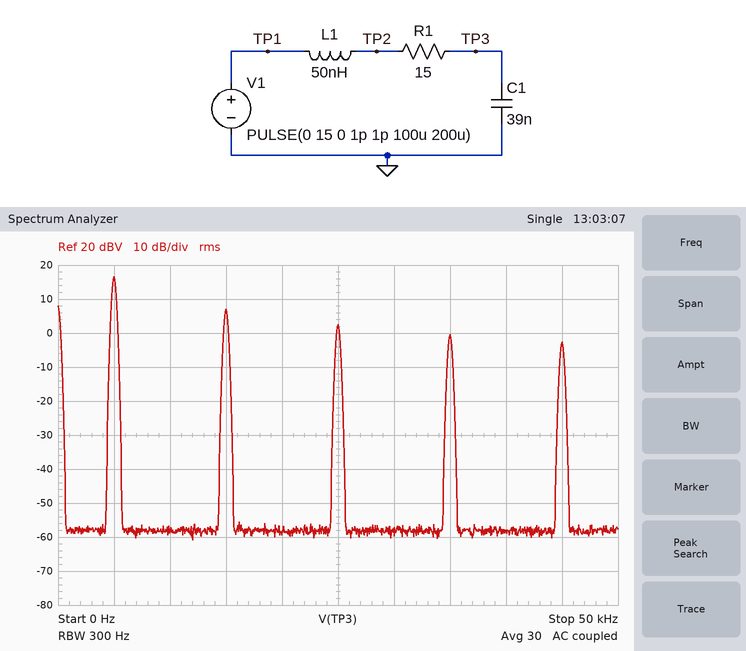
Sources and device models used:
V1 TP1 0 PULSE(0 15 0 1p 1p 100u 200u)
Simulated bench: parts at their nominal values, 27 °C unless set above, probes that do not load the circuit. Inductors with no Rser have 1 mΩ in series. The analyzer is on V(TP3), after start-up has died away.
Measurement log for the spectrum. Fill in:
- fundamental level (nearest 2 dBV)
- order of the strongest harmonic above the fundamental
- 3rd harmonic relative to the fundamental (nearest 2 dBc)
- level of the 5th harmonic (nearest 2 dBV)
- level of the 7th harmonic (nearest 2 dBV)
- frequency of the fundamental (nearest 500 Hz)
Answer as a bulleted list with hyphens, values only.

- 16 dBV
- 3
- -10 dBc
- 2 dBV
- 0 dBV
- 5.0 kHz
